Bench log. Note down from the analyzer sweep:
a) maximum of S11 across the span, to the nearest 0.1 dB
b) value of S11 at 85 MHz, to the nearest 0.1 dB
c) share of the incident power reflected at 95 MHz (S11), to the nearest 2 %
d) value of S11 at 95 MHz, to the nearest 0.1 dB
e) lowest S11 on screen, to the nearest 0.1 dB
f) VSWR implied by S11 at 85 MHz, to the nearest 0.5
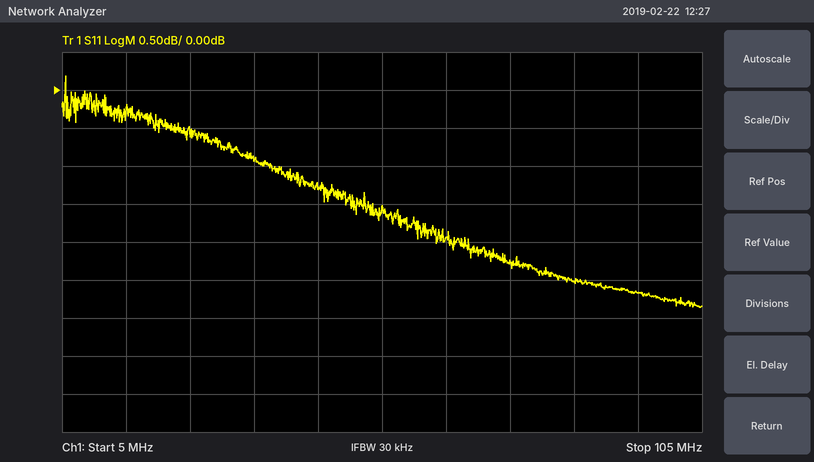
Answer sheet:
0.2 dB
-2.5 dB
54 %
-2.7 dB
-2.9 dB
7.0
